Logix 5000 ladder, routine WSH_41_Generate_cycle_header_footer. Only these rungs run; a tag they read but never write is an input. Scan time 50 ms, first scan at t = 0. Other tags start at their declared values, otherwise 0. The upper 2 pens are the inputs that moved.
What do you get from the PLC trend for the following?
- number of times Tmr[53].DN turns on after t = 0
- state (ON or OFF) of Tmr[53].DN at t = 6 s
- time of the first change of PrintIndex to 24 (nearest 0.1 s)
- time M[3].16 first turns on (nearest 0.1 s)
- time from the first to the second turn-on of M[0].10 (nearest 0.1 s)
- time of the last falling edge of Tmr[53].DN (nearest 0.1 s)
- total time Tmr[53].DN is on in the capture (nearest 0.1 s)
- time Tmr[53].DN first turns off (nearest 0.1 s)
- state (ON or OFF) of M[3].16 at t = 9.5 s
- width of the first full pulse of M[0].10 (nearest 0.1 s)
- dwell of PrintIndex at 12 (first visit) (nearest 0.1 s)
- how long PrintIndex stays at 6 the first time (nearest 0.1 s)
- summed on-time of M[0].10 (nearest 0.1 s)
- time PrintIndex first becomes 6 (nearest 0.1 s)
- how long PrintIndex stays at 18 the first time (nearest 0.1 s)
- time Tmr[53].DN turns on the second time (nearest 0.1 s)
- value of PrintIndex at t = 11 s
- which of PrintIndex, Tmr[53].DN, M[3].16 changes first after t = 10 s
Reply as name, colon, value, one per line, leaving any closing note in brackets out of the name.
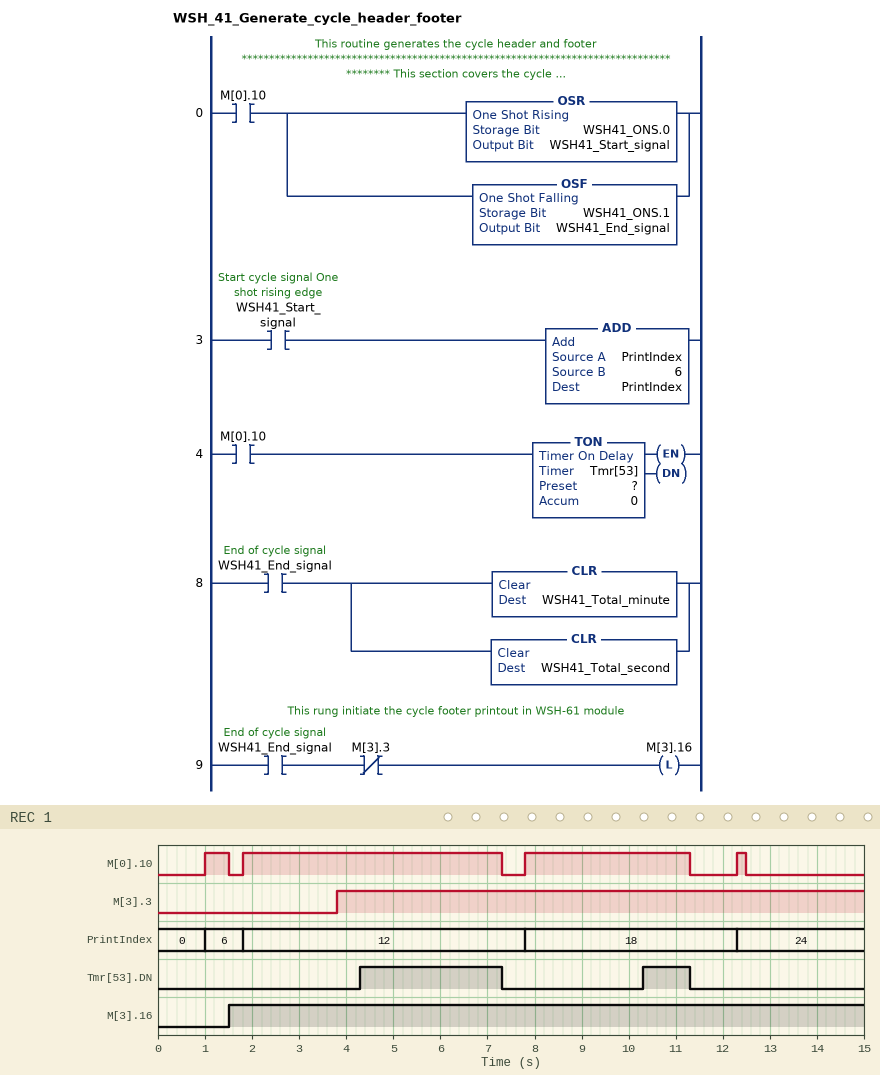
number of times Tmr[53].DN turns on after t = 0: 2
state (ON or OFF) of Tmr[53].DN at t = 6 s: ON
time of the first change of PrintIndex to 24: 12.3 s
time M[3].16 first turns on: 1.5 s
time from the first to the second turn-on of M[0].10: 0.8 s
time of the last falling edge of Tmr[53].DN: 11.3 s
total time Tmr[53].DN is on in the capture: 4.0 s
time Tmr[53].DN first turns off: 7.3 s
state (ON or OFF) of M[3].16 at t = 9.5 s: ON
width of the first full pulse of M[0].10: 0.5 s
dwell of PrintIndex at 12 (first visit): 6.0 s
how long PrintIndex stays at 6 the first time: 0.8 s
summed on-time of M[0].10: 9.7 s
time PrintIndex first becomes 6: 1.0 s
how long PrintIndex stays at 18 the first time: 4.5 s
time Tmr[53].DN turns on the second time: 10.3 s
value of PrintIndex at t = 11 s: 18
which of PrintIndex, Tmr[53].DN, M[3].16 changes first after t = 10 s: Tmr[53].DN
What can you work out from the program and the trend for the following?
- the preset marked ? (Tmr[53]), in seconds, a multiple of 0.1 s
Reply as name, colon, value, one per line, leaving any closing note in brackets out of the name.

the preset marked ? (Tmr[53]), in seconds, a multiple of 0.1 s: 2.5 s
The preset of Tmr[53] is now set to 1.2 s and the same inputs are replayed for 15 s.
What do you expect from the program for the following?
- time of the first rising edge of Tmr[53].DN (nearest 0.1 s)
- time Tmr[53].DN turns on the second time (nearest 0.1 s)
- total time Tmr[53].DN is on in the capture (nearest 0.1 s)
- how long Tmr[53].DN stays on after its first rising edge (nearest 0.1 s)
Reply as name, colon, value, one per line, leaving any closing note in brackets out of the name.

time of the first rising edge of Tmr[53].DN: 3.0 s
time Tmr[53].DN turns on the second time: 9.0 s
total time Tmr[53].DN is on in the capture: 6.6 s
how long Tmr[53].DN stays on after its first rising edge: 4.3 s
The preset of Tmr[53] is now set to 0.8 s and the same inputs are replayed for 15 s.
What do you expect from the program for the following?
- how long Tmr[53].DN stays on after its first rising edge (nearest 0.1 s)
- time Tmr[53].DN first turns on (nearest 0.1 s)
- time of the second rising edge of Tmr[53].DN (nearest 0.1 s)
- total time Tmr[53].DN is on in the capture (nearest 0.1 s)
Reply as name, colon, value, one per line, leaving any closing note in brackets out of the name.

how long Tmr[53].DN stays on after its first rising edge: 4.7 s
time Tmr[53].DN first turns on: 2.6 s
time of the second rising edge of Tmr[53].DN: 8.6 s
total time Tmr[53].DN is on in the capture: 7.4 s
